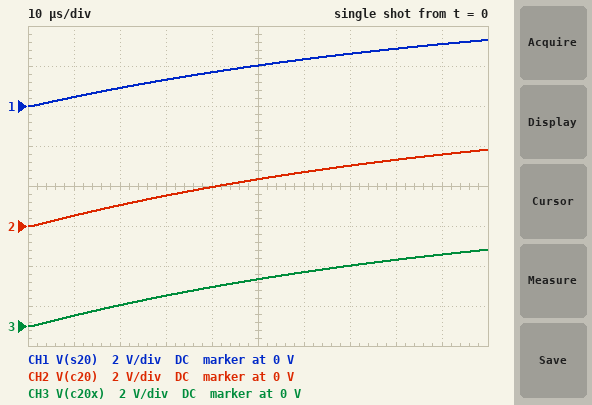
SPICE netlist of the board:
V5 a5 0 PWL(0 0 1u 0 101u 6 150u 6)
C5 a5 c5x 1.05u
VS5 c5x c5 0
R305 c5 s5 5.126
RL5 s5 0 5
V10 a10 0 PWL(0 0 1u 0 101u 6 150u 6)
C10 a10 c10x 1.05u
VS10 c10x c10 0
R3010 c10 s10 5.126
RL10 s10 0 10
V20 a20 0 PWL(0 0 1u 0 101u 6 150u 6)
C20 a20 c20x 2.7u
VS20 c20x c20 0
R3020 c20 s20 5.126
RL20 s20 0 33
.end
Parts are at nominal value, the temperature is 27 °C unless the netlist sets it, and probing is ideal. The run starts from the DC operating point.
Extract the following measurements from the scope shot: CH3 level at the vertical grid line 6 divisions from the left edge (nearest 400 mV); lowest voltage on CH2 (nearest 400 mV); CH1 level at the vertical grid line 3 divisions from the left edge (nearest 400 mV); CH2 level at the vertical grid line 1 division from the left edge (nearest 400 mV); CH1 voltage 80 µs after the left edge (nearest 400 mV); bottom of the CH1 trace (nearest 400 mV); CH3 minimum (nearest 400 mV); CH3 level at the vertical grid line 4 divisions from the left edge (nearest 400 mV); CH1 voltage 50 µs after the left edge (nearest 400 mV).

2.8 V
0 V
1.2 V
400 mV
2.8 V
0 V
0 V
2.0 V
2.0 V
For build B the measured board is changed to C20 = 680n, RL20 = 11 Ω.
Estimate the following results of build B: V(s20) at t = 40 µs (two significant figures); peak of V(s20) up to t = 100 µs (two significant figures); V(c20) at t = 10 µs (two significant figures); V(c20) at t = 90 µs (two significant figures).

440 mV
450 mV
370 mV
660 mV
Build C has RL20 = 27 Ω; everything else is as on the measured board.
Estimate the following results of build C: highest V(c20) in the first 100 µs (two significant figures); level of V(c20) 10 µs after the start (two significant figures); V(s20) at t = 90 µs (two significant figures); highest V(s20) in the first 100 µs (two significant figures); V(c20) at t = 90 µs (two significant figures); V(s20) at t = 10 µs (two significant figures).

3.5 V
510 mV
2.8 V
3.0 V
3.3 V
430 mV
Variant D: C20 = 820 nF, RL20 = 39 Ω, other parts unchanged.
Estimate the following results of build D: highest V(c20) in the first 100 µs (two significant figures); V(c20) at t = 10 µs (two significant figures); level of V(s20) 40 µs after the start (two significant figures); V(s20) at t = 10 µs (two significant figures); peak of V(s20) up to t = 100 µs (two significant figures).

2.0 V
480 mV
1.3 V
420 mV
1.8 V
